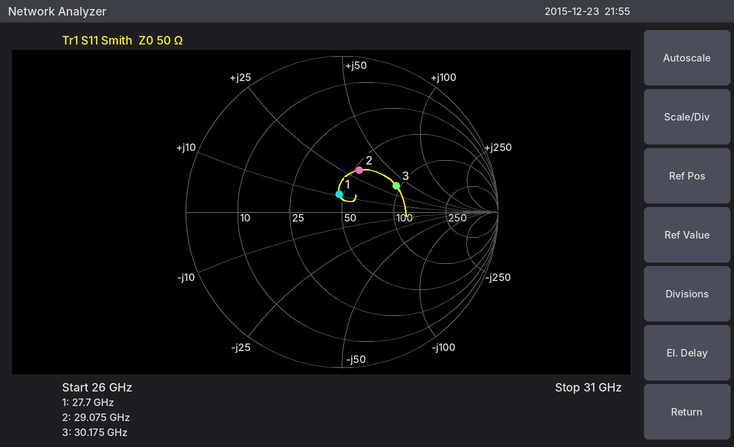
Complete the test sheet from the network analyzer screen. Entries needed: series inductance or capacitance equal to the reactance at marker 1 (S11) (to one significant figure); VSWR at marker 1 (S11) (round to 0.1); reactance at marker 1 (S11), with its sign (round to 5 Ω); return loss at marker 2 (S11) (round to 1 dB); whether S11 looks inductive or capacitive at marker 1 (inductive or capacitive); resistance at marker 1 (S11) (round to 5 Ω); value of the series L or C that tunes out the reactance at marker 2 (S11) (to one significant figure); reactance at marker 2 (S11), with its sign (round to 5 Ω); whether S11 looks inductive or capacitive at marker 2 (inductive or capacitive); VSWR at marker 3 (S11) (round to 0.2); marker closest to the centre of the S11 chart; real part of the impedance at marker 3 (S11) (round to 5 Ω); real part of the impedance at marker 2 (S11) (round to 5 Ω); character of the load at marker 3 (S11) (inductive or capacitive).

60 pH
1.3
+10 Ω
11 dB
inductive
45 Ω
200 fF
+30 Ω
inductive
2.2
marker 1
95 Ω
55 Ω
inductive
